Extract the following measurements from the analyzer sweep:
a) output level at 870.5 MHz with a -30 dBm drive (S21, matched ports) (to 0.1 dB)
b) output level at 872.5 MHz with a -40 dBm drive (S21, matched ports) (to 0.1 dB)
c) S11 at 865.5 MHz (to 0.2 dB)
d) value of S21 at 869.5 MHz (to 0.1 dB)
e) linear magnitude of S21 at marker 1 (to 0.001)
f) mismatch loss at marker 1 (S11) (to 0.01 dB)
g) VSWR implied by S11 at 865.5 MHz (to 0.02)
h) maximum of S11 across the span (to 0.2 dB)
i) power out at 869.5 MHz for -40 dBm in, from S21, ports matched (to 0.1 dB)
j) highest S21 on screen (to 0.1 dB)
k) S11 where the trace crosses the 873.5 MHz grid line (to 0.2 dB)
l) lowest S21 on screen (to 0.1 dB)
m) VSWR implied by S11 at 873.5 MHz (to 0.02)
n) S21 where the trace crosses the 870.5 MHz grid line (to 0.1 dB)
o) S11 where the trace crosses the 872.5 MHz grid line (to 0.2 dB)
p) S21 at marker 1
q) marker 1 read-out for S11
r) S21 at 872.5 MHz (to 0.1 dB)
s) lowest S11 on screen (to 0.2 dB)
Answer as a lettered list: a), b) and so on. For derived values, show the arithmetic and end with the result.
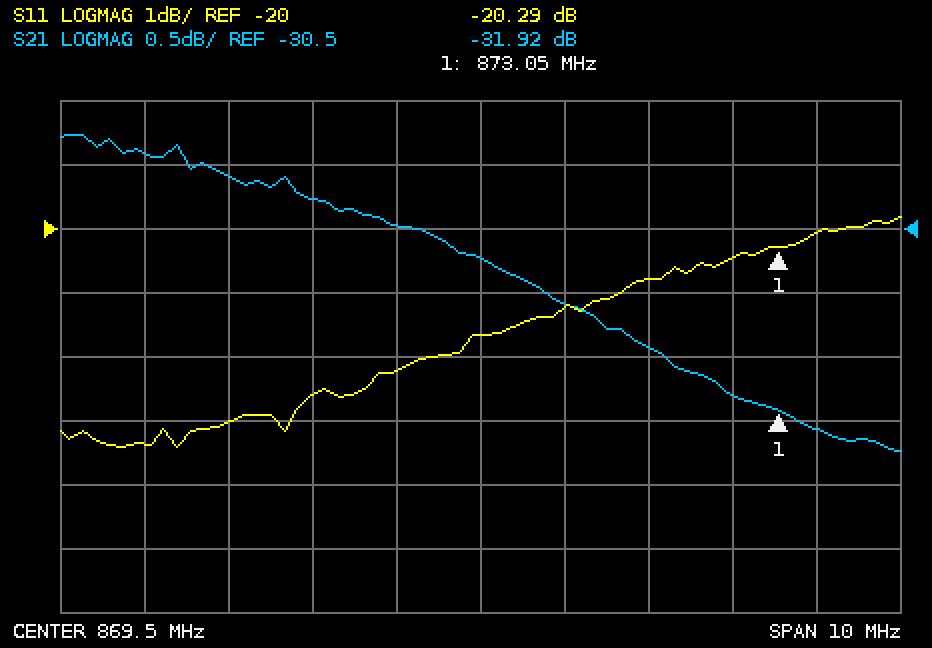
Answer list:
a) -30 dBm + (-31.1 dB) = -61.1 dBm
b) -40 dBm + (-31.8 dB) = -71.8 dBm
c) -23.4 dB
d) -30.7 dB
e) 10^(-31.92/20) ≈ 0.025
f) −10 log10(1 − 10^(-20.29/10)) ≈ 0.04 dB
g) |Γ| = 10^(-23.4/20) = 0.0676; VSWR = (1 + 0.0676)/(1 − 0.0676) ≈ 1.15, so 1.14 to the nearest 0.02
h) -19.8 dB
i) -40 dBm + (-30.7 dB) = -70.7 dBm
j) -29.8 dB
k) -20.0 dB
l) -32.2 dB
m) |Γ| = 10^(-20/20) = 0.1000; VSWR = (1 + 0.1000)/(1 − 0.1000) ≈ 1.22
n) -31.1 dB
o) -20.4 dB
p) -31.92 dB
q) -20.29 dB
r) -31.8 dB
s) -23.4 dB
